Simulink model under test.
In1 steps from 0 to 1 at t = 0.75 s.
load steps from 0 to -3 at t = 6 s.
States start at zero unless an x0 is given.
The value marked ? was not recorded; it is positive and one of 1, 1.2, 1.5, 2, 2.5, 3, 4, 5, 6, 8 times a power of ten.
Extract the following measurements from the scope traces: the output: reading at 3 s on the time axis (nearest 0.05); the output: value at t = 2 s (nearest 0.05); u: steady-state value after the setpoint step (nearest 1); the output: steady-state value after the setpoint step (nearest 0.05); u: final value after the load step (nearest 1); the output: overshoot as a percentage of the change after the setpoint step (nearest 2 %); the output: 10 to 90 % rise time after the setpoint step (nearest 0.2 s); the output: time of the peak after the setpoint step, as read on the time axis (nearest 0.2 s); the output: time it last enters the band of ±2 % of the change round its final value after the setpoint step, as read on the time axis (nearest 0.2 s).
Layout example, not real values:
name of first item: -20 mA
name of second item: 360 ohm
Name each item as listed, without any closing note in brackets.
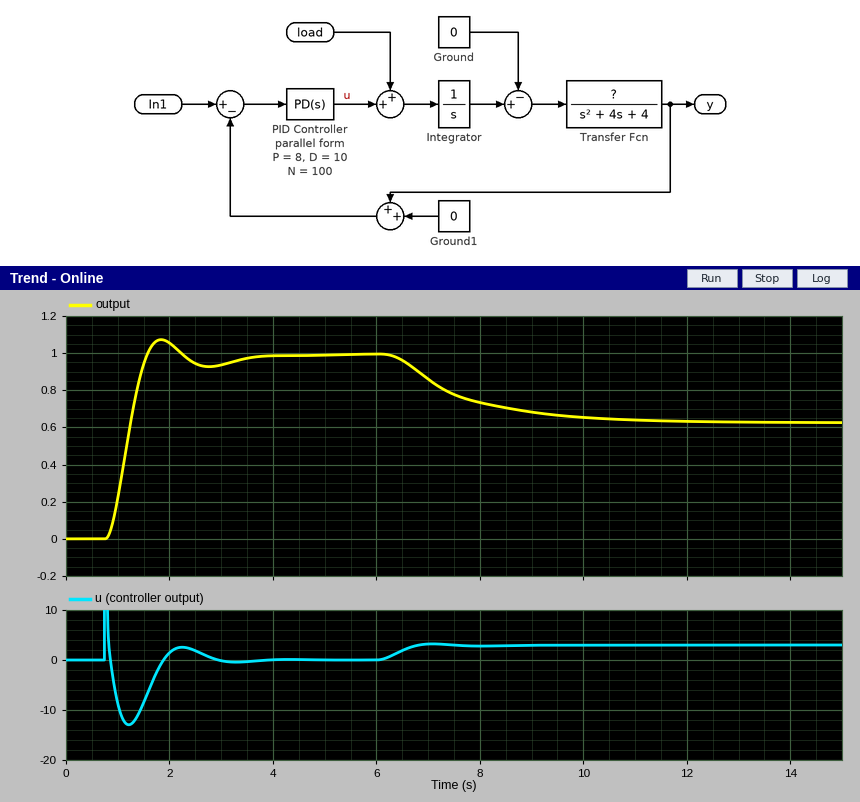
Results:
the output: reading at 3 s on the time axis: 0.95
the output: value at t = 2 s: 1.05
u: steady-state value after the setpoint step: 0
the output: steady-state value after the setpoint step: 1.00
u: final value after the load step: 3
the output: overshoot as a percentage of the change after the setpoint step: 8 %
the output: 10 to 90 % rise time after the setpoint step: 0.6 s
the output: time of the peak after the setpoint step, as read on the time axis: 1.8 s
the output: time it last enters the band of ±2 % of the change round its final value after the setpoint step, as read on the time axis: 3.6 s
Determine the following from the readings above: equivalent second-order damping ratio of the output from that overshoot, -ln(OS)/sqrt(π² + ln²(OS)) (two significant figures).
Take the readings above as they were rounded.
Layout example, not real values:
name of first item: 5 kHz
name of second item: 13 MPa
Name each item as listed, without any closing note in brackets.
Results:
equivalent second-order damping ratio of the output from that overshoot, -ln(OS)/sqrt(π² + ln²(OS)): 0.63
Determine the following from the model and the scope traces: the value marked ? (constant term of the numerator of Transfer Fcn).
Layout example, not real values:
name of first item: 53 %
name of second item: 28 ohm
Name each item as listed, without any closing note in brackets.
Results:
the value marked ?: 1
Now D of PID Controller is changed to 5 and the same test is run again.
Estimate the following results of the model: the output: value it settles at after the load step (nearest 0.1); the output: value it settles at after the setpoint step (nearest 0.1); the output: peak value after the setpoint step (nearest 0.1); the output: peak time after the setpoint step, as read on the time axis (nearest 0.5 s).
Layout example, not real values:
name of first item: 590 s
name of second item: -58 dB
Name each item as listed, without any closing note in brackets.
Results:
the output: value it settles at after the load step: 0.6
the output: value it settles at after the setpoint step: 1.0
the output: peak value after the setpoint step: 1.1
the output: peak time after the setpoint step, as read on the time axis: 2.5 s
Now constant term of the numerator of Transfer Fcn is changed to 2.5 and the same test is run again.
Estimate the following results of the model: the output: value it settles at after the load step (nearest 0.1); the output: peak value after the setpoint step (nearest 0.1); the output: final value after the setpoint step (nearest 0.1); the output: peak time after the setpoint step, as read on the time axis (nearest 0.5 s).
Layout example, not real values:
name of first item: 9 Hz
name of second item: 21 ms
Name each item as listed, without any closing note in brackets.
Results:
the output: value it settles at after the load step: 0.6
the output: peak value after the setpoint step: 1.3
the output: final value after the setpoint step: 1.0
the output: peak time after the setpoint step, as read on the time axis: 1.5 s
